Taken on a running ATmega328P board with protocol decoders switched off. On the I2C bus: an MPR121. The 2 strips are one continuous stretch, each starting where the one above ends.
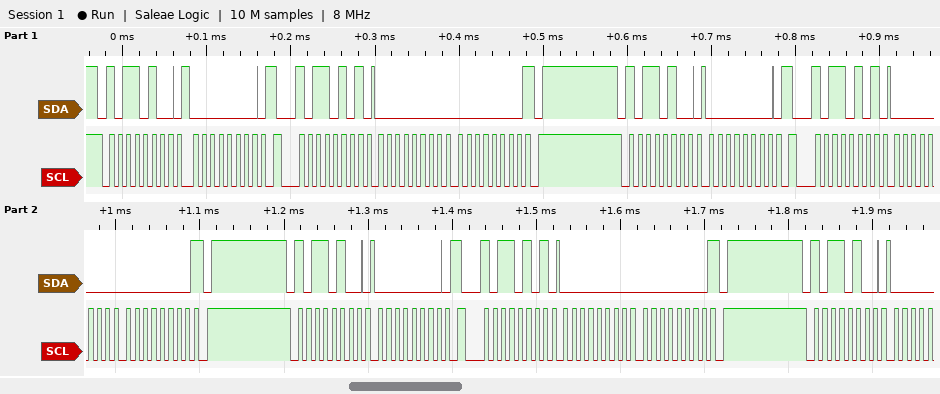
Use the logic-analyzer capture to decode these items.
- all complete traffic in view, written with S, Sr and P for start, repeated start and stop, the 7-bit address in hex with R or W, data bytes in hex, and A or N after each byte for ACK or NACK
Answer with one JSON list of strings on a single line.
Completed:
["S 5AW A 00 A Sr 5AR A 00 A 00 N P S 5AW A 00 A Sr 5AR A 00 A 00 N P S 5AW A 00 A Sr 5AR A 00 A 00 N P S 5AW A"]
